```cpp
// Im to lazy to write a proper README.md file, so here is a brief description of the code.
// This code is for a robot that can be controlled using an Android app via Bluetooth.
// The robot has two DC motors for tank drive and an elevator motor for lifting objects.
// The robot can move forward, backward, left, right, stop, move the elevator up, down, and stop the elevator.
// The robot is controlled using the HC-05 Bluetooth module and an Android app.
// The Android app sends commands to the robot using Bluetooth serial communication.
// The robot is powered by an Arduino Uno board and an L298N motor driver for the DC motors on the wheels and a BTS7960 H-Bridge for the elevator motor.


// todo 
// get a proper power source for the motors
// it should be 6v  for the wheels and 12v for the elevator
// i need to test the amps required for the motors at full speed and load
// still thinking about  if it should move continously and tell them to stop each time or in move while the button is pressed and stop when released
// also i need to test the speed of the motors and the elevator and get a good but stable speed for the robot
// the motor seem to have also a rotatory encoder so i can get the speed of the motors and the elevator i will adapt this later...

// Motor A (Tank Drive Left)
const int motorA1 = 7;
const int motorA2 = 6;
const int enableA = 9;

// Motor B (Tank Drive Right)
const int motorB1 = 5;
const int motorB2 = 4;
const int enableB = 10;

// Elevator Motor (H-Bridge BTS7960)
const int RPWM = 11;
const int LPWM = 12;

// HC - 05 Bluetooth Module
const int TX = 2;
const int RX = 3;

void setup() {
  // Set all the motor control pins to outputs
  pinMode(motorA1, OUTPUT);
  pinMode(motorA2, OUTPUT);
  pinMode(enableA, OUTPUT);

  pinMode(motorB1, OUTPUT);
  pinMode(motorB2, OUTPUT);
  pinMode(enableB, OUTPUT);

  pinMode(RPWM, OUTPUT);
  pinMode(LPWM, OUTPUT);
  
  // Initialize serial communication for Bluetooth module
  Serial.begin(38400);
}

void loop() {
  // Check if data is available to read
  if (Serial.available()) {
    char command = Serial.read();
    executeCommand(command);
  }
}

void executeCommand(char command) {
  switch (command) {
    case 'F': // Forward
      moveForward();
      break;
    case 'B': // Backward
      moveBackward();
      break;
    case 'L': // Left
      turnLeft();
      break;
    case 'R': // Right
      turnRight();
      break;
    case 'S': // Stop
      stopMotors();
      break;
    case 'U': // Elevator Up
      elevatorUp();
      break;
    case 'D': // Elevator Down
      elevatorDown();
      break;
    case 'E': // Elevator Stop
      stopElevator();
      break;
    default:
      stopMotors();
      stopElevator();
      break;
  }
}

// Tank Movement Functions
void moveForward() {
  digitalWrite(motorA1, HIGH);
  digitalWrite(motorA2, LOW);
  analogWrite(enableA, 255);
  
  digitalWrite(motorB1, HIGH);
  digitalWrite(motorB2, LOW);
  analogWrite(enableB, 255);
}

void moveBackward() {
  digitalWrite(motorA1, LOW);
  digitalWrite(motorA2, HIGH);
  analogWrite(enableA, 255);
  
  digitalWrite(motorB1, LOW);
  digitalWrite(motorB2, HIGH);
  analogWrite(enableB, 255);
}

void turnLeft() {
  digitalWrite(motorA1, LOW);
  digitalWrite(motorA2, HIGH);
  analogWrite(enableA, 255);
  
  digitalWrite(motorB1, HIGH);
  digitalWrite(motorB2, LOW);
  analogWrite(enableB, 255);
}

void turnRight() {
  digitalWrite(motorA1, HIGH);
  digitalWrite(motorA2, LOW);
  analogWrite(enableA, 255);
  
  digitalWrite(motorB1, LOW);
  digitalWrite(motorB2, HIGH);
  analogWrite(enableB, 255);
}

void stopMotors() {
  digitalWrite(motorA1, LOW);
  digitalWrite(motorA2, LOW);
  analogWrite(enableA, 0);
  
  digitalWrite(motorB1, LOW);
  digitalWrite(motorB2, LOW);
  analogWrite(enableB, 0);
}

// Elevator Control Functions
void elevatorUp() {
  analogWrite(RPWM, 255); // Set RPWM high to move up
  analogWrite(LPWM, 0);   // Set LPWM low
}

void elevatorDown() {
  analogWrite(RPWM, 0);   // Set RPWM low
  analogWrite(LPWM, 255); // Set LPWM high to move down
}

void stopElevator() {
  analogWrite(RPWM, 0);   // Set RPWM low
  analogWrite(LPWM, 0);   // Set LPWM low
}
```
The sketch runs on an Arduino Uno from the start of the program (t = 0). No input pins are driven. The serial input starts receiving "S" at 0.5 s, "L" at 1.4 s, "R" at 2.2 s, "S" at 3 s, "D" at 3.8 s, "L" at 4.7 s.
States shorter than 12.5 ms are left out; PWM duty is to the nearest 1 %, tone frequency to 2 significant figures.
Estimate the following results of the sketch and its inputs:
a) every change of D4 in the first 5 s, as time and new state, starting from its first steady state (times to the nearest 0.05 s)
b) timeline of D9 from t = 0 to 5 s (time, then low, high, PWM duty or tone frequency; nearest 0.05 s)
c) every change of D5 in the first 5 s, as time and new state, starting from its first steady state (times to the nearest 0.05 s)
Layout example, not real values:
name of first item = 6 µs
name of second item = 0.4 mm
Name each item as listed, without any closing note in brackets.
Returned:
every change of D4 in the first 5 s, as time and new state, starting from its first steady state = 0 s low; 2.2 s high; 3 s low
timeline of D9 from t = 0 to 5 s = 0 s low; 1.4 s high; 3 s low; 4.7 s high
every change of D5 in the first 5 s, as time and new state, starting from its first steady state = 0 s low; 1.4 s high; 2.2 s low; 4.7 s high
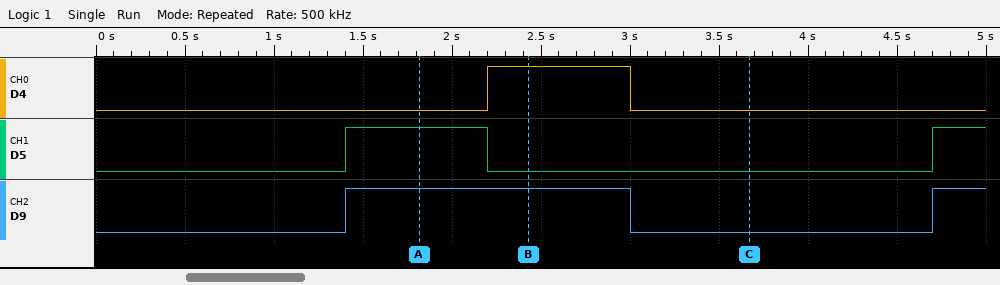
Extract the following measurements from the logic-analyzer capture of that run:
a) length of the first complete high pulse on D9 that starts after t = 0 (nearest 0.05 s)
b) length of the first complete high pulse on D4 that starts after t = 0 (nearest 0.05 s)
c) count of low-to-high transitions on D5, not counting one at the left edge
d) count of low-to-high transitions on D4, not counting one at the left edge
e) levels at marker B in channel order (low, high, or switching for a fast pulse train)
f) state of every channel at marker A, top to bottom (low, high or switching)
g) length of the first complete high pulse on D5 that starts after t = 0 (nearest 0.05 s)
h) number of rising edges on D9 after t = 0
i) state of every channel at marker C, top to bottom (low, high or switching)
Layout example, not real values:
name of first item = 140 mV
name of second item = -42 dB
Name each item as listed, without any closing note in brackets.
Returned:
length of the first complete high pulse on D9 that starts after t = 0 = 1.60 s
length of the first complete high pulse on D4 that starts after t = 0 = 0.80 s
count of low-to-high transitions on D5, not counting one at the left edge = 2
count of low-to-high transitions on D4, not counting one at the left edge = 1
levels at marker B in channel order = D4 high, D5 low, D9 high
state of every channel at marker A, top to bottom = D4 low, D5 high, D9 high
length of the first complete high pulse on D5 that starts after t = 0 = 0.80 s
number of rising edges on D9 after t = 0 = 2
state of every channel at marker C, top to bottom = D4 low, D5 low, D9 low
